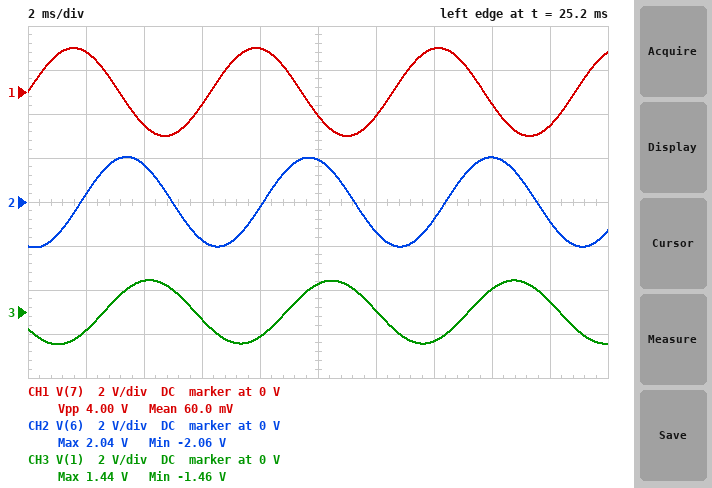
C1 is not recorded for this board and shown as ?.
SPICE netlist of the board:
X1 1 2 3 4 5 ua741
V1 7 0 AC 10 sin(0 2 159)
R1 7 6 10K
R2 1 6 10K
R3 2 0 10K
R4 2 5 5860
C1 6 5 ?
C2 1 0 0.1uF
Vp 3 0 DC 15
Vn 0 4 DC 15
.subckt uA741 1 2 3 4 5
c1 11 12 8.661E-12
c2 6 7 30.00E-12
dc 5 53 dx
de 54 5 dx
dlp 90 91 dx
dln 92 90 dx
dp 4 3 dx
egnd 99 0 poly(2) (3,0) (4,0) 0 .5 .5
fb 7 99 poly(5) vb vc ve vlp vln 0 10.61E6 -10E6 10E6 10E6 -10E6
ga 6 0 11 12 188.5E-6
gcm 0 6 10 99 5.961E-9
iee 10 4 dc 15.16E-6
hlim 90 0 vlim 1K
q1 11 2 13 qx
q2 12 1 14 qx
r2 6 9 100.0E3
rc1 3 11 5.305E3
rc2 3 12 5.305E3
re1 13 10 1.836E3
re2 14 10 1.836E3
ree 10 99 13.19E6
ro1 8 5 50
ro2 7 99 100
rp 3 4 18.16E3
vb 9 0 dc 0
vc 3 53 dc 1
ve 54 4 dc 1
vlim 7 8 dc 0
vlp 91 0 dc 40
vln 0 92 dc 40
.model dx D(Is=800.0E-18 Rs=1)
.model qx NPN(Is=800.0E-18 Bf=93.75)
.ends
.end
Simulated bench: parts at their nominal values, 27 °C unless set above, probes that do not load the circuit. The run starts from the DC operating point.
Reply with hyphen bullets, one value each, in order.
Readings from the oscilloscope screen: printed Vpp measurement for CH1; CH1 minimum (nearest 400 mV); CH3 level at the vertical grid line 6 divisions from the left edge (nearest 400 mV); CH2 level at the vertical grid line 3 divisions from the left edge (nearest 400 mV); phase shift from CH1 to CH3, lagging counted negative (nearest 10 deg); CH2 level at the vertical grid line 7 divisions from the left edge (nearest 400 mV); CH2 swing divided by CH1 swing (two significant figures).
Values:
- 4.00 V
- -2.0 V
- 0 V
- -1.6 V
- -150 deg
- -800 mV
- 1.0
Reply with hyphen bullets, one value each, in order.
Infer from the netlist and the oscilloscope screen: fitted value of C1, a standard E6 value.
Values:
- 220 nF
